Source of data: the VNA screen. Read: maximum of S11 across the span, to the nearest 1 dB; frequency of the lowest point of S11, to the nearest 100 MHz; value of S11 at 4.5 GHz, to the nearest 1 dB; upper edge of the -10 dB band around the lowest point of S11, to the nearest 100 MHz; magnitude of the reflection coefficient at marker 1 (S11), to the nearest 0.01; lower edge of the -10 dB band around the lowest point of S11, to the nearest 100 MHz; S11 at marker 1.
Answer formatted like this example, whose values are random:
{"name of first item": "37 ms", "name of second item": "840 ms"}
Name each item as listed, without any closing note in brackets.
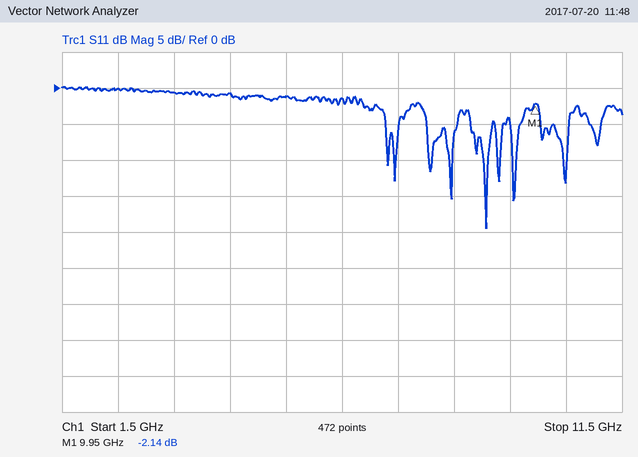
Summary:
{"maximum of S11 across the span, to the nearest 1 dB": "0 dB", "frequency of the lowest point of S11, to the nearest 100 MHz": "9.1 GHz", "value of S11 at 4.5 GHz, to the nearest 1 dB": "-1 dB", "upper edge of the -10 dB band around the lowest point of S11, to the nearest 100 MHz": "9.1 GHz", "magnitude of the reflection coefficient at marker 1 (S11), to the nearest 0.01": "0.78", "lower edge of the -10 dB band around the lowest point of S11, to the nearest 100 MHz": "9.0 GHz", "S11 at marker 1": "-2.14 dB"}
